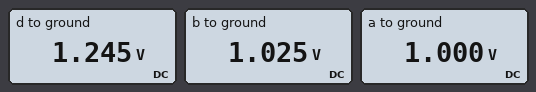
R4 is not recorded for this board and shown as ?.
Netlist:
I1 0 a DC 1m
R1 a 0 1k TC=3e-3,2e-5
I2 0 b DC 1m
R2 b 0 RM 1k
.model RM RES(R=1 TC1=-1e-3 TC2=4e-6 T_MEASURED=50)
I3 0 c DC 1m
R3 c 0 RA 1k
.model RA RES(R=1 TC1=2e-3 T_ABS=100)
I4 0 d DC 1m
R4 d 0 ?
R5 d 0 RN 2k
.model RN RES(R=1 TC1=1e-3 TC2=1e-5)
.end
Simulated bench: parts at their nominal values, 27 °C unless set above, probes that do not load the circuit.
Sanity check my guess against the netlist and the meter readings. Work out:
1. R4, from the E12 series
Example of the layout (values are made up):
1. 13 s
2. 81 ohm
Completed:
1. 3.3 kΩ
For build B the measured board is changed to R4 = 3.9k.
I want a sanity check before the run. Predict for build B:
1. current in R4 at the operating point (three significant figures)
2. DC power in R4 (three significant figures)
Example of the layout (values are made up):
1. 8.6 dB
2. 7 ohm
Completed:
1. 339 µA
2. 448 µW
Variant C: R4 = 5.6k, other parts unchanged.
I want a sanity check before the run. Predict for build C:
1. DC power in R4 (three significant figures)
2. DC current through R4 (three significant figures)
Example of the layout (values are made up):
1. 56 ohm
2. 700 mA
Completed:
1. 388 µW
2. 263 µA
